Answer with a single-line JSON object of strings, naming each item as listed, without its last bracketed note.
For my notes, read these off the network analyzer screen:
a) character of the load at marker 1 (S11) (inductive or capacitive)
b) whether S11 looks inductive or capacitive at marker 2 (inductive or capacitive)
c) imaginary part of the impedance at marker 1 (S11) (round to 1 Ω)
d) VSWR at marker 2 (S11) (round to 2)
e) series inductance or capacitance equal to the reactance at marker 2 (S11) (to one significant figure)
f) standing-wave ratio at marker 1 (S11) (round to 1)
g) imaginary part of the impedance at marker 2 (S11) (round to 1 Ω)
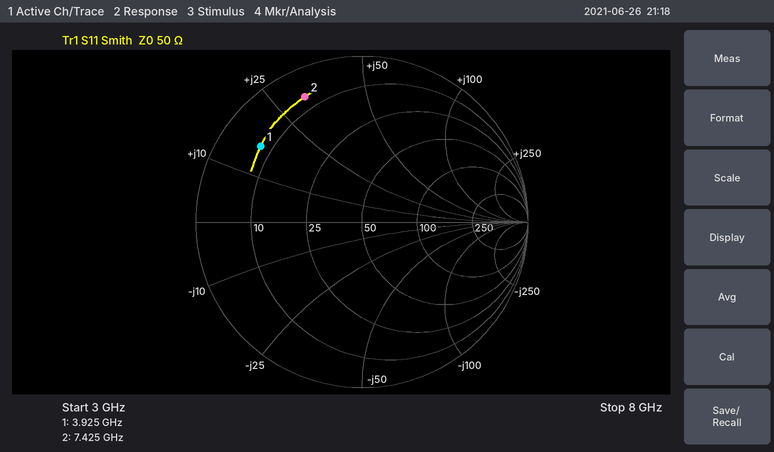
{"character of the load at marker 1 (S11)": "inductive", "whether S11 looks inductive or capacitive at marker 2": "inductive", "imaginary part of the impedance at marker 1 (S11)": "+16 Ω", "VSWR at marker 2 (S11)": "10", "series inductance or capacitance equal to the reactance at marker 2 (S11)": "700 pH", "standing-wave ratio at marker 1 (S11)": "7", "imaginary part of the impedance at marker 2 (S11)": "+32 Ω"}
